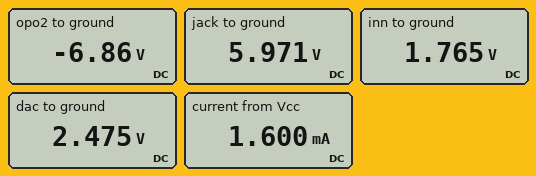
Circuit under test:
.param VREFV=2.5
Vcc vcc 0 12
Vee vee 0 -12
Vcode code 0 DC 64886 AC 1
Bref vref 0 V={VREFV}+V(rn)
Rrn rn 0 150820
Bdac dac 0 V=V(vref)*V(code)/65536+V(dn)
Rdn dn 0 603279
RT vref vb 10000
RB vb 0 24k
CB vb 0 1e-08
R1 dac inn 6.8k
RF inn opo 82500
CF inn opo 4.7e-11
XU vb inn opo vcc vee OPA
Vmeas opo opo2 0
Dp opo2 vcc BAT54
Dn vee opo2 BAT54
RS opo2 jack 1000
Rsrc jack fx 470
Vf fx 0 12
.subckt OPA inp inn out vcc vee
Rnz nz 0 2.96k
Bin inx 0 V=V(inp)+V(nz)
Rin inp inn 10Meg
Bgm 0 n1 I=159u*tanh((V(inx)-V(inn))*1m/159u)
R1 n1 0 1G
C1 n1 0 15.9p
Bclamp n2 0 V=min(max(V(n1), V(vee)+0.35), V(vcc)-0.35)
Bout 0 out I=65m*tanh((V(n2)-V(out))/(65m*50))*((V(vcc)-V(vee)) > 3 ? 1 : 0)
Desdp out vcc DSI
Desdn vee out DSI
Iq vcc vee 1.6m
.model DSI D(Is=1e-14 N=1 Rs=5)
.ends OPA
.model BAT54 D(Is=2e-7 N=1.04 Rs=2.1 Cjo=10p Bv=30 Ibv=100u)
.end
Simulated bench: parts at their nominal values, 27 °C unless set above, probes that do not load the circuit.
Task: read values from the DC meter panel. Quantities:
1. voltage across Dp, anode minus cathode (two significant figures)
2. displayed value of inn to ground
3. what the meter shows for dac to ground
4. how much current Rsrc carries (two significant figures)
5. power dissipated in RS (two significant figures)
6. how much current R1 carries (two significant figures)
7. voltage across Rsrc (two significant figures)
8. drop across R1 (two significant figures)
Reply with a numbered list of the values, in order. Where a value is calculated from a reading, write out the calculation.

1. -6.86 V - 12 V = -19 V
2. 1.765 V
3. 2.475 V
4. (12 V - 5.971 V) / 470 Ω = 13 mA
5. (5.971 V - (-6.86 V))^2 / 1 kΩ = 160 mW
6. (2.475 V - 1.765 V) / 6.8 kΩ = 100 µA
7. 12 V - 5.971 V = 6.0 V
8. 2.475 V - 1.765 V = 710 mV
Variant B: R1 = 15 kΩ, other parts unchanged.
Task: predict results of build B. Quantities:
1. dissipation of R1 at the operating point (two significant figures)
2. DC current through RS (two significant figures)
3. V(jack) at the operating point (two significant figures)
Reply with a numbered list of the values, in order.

1. 34 µW
2. 9.6 mA
3. 7.5 V
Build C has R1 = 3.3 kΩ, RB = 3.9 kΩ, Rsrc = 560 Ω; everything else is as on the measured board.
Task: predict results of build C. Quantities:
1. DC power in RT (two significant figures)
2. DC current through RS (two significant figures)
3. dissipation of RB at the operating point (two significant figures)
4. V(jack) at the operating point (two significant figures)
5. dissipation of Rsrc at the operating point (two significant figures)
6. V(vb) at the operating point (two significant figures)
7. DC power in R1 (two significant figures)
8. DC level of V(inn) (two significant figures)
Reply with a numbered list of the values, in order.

1. 320 µW
2. 15 mA
3. 130 µW
4. 3.8 V
5. 120 mW
6. 700 mV
7. 80 µW
8. 2.0 V
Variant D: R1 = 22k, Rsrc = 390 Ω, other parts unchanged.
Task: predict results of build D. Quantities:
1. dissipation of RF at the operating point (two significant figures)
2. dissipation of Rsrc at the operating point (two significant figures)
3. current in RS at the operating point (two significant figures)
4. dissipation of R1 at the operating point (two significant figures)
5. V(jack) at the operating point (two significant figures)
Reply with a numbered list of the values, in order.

1. 86 µW
2. 34 mW
3. 9.3 mA
4. 23 µW
5. 8.4 V
